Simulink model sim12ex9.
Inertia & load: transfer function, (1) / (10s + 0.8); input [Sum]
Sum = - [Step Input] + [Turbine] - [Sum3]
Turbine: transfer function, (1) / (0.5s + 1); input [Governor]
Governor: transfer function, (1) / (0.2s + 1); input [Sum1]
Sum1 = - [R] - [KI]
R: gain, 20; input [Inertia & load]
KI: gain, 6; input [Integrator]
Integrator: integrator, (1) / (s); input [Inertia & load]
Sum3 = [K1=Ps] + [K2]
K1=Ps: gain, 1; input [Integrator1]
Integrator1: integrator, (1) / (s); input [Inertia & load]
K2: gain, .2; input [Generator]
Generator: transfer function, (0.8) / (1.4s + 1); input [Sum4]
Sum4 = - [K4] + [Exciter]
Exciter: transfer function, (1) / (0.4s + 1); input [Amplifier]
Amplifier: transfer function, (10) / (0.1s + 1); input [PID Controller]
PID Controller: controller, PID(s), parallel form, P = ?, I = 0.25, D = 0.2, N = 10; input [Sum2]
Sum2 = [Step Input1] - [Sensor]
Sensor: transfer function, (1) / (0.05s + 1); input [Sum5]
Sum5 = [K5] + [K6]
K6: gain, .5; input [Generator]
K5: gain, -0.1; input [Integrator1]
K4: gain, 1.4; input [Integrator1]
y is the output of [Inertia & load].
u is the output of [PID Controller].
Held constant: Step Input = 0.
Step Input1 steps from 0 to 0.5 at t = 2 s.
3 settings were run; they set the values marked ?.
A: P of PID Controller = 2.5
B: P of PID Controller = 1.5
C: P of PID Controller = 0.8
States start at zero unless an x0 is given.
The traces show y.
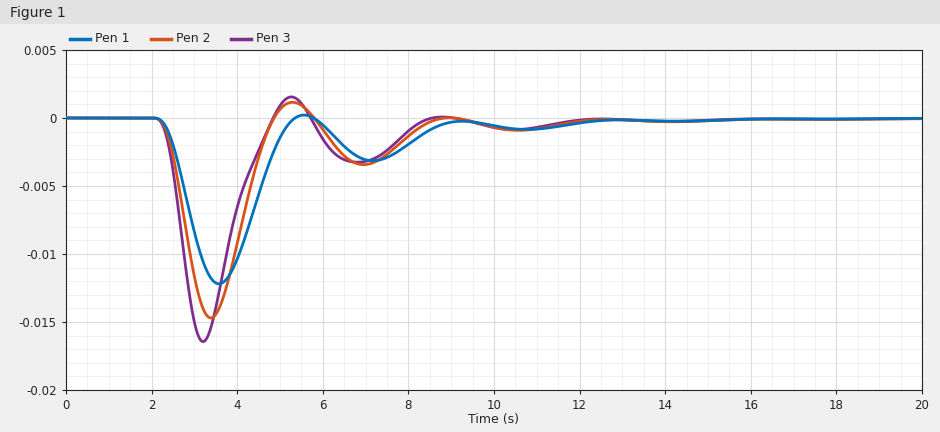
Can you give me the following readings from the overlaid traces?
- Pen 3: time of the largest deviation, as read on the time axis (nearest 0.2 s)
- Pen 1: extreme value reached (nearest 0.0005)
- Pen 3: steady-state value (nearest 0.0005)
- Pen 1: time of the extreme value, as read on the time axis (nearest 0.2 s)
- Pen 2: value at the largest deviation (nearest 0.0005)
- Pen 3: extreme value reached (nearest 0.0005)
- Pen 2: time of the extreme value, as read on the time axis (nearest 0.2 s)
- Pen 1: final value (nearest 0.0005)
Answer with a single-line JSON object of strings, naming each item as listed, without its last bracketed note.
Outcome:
{"Pen 3: time of the largest deviation, as read on the time axis": "3.2 s", "Pen 1: extreme value reached": "-0.0120", "Pen 3: steady-state value": "0.0000", "Pen 1: time of the extreme value, as read on the time axis": "3.6 s", "Pen 2: value at the largest deviation": "-0.0145", "Pen 3: extreme value reached": "-0.0165", "Pen 2: time of the extreme value, as read on the time axis": "3.4 s", "Pen 1: final value": "0.0000"}
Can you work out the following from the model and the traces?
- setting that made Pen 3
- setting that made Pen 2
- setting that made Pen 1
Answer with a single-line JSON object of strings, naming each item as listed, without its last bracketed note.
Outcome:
{"setting that made Pen 3": "A", "setting that made Pen 2": "B", "setting that made Pen 1": "C"}
